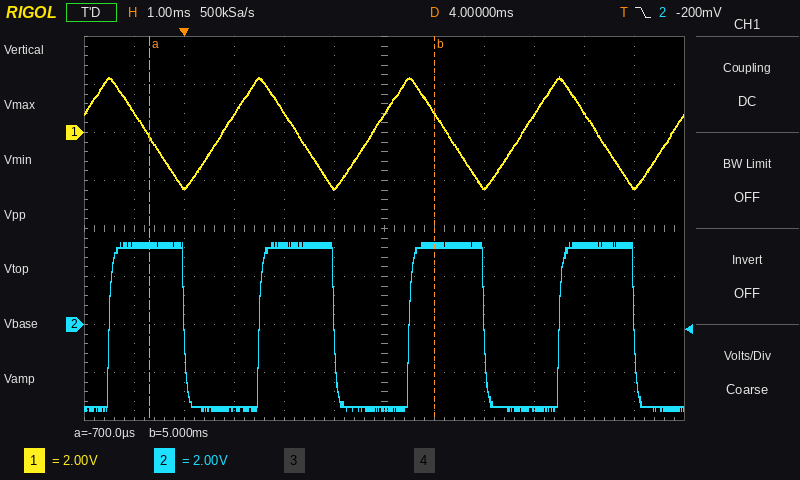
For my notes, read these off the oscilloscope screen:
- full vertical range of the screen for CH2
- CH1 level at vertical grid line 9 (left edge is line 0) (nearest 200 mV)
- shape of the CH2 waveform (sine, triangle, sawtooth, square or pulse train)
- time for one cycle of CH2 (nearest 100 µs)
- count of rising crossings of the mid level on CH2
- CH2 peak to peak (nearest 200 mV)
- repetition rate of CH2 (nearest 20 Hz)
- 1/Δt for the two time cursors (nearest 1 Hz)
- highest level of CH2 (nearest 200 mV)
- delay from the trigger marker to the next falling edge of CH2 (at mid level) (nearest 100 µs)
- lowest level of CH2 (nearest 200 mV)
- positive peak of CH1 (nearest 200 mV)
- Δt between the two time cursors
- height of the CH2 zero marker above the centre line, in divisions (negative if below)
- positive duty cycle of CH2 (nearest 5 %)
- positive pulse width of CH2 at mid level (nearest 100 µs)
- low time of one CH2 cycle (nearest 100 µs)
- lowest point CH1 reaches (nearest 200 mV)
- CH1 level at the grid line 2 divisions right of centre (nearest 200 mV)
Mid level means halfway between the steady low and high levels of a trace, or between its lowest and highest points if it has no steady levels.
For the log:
16 V
800 mV
square
3.0 ms
4
7.0 V
340 Hz
175 Hz
3.4 V
3.0 ms
-3.6 V
2.4 V
5.7 ms
-2.0 div
50 %
1.5 ms
1.5 ms
-2.4 V
-2.2 V
